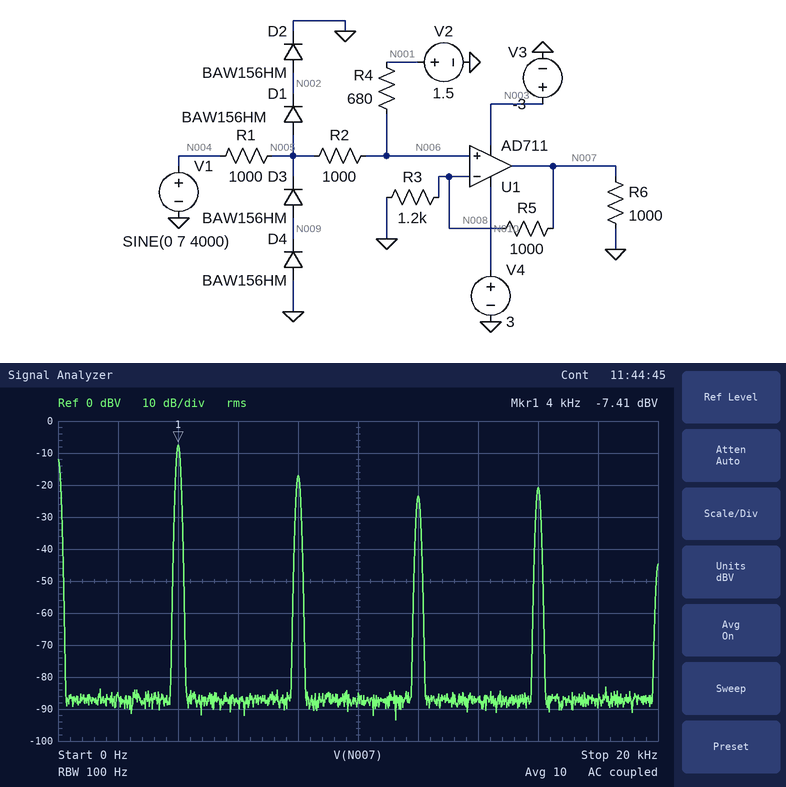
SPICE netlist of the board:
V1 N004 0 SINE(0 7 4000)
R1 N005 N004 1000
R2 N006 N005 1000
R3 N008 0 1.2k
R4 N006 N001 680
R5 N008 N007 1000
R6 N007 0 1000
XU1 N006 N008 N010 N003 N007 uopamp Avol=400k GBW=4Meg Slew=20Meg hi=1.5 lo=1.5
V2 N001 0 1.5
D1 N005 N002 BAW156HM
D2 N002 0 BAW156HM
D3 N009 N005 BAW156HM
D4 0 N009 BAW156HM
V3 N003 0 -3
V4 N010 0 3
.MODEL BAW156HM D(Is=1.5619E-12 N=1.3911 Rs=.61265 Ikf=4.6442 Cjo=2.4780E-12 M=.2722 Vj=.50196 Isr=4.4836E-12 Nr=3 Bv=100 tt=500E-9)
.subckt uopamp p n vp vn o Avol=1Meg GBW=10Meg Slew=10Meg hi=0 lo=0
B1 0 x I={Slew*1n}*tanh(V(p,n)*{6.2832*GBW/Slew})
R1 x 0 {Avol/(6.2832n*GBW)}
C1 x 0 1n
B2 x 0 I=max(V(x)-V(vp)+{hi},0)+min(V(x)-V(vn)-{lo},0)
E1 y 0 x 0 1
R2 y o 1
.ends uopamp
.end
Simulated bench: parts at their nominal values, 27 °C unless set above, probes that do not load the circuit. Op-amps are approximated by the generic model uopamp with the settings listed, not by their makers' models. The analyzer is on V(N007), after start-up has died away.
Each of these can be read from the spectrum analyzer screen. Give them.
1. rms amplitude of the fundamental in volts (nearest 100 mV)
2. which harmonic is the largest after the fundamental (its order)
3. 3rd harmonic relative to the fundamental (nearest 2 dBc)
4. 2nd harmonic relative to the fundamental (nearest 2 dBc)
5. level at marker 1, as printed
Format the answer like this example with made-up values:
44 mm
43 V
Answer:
400 mV
2
-16 dBc
-10 dBc
-7.41 dBV
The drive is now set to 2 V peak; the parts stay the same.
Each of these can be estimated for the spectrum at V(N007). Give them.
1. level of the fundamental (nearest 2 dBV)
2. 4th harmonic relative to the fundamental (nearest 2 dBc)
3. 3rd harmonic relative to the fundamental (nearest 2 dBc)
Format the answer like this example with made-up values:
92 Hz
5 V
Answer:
-20 dBV
-16 dBc
-8 dBc
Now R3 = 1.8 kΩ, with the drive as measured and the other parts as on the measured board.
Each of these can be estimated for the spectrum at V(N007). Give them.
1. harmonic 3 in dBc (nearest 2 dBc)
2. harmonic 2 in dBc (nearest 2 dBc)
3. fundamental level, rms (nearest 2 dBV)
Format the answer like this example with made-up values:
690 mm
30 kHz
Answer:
-14 dBc
-10 dBc
-6 dBV
